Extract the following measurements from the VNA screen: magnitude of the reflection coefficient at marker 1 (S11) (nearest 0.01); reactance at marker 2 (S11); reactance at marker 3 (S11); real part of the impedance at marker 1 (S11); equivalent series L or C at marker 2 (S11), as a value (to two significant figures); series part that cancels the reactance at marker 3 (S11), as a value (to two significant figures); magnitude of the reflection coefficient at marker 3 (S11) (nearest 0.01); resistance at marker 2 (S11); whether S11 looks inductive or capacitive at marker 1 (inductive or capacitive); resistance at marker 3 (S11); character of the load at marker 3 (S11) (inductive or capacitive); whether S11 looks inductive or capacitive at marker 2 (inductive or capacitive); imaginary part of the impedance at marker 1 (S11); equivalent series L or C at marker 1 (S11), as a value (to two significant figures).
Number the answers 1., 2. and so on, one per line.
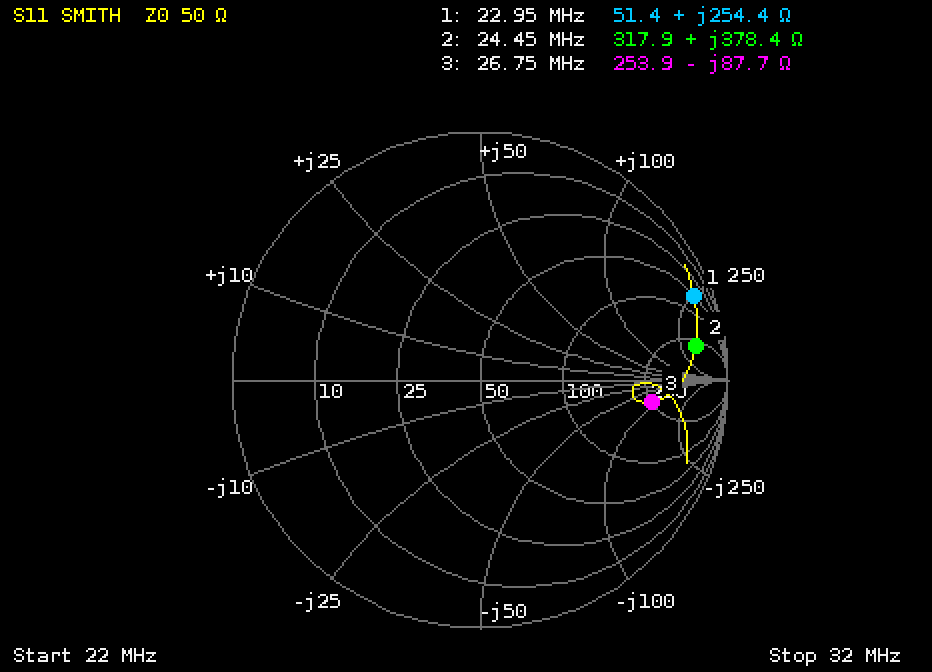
1. 0.93
2. +378.4 Ω
3. -87.7 Ω
4. 51.4 Ω
5. 2.5 µH
6. 520 nH
7. 0.70
8. 317.9 Ω
9. inductive
10. 253.9 Ω
11. capacitive
12. inductive
13. +254.4 Ω
14. 1.8 µH
